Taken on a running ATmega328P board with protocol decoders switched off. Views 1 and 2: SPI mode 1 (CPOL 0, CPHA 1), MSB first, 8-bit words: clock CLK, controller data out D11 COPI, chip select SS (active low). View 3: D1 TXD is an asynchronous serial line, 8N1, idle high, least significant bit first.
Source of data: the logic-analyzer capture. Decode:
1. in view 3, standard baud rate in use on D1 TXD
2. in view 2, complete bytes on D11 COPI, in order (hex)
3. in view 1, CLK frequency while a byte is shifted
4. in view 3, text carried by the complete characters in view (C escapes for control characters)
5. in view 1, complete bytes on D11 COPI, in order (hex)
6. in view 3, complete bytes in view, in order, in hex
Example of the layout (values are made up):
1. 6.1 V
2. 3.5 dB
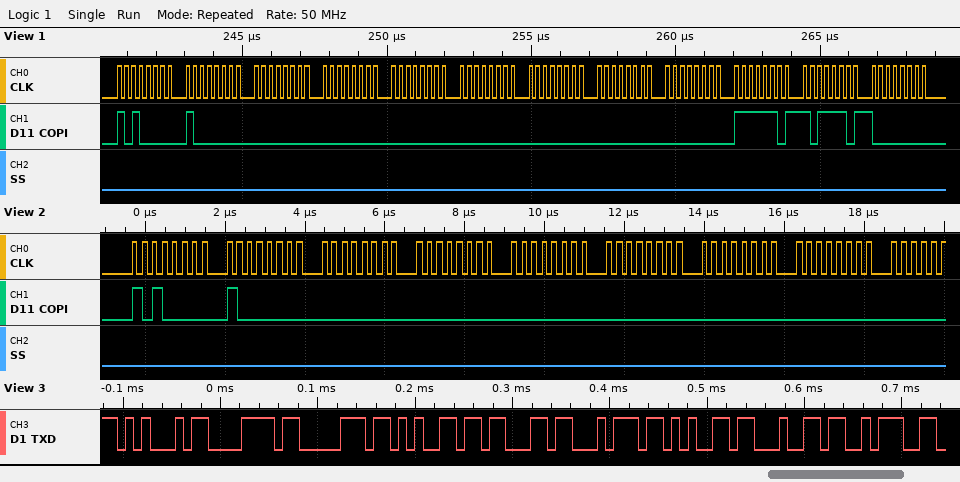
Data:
1. 115200 baud
2. A0 80 00 00 00 00 00 00
3. 4 MHz
4. "Expected:"
5. A0 80 00 00 00 00 00 00 00 FD BD 00
6. 45 78 70 65 63 74 65 64 3A
